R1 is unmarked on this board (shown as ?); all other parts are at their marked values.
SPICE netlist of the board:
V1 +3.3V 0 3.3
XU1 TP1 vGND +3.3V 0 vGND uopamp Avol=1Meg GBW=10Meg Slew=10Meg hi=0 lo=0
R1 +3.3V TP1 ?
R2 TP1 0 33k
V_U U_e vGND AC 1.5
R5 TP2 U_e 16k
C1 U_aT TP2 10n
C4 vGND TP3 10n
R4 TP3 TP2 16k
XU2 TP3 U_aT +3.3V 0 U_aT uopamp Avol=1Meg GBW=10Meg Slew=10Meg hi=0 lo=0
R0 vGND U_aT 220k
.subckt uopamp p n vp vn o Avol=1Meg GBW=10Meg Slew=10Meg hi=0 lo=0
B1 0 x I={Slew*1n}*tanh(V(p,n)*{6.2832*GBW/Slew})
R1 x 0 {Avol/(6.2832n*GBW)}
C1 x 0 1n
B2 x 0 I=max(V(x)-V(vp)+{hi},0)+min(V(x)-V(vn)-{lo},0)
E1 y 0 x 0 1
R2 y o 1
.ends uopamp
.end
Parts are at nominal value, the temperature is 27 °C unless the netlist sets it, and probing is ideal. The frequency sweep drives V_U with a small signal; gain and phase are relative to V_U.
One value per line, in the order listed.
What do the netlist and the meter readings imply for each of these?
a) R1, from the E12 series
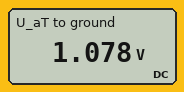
68 kΩ
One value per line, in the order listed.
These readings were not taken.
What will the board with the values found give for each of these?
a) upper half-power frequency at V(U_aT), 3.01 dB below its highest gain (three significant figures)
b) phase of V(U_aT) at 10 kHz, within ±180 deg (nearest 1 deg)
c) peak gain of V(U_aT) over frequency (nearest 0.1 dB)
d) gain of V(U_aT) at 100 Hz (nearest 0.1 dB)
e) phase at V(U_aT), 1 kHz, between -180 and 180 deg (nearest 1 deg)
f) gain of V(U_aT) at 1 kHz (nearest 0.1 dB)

640 Hz
-169 deg
0 dB
-0.1 dB
-90 deg
-6.1 dB
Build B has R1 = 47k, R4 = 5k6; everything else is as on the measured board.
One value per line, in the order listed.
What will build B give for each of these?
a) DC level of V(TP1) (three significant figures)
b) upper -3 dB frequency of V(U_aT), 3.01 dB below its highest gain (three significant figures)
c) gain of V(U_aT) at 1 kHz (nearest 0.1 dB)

1.36 V
900 Hz
-3.5 dB
